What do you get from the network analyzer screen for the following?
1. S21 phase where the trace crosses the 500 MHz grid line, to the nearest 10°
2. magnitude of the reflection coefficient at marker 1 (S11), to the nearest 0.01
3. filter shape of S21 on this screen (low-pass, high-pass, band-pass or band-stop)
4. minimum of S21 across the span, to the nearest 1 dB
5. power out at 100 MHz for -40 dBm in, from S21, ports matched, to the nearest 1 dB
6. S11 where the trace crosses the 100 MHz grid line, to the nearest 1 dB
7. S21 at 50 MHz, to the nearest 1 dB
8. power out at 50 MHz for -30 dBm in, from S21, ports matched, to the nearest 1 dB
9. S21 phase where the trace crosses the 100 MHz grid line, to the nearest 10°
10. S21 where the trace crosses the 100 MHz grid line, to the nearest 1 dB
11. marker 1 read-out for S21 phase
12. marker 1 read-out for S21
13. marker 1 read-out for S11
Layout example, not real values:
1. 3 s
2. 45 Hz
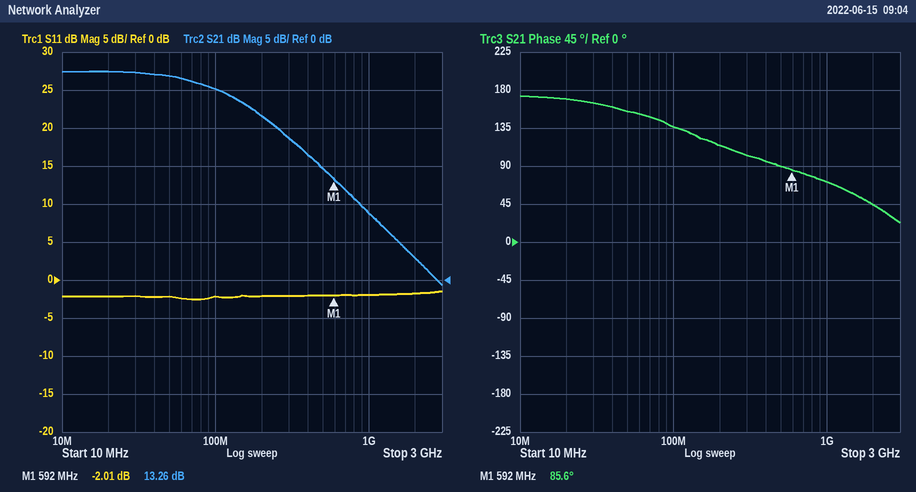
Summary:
1. 90°
2. 0.79
3. low-pass
4. -1 dB
5. -15 dBm
6. -2 dB
7. 27 dB
8. -3 dBm
9. 140°
10. 25 dB
11. 85.6°
12. 13.26 dB
13. -2.01 dB
